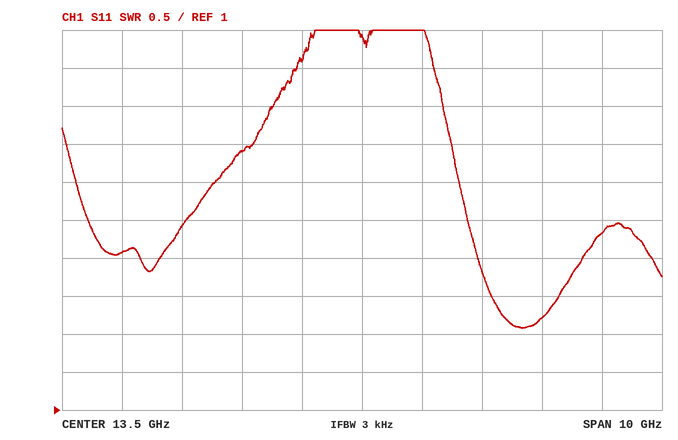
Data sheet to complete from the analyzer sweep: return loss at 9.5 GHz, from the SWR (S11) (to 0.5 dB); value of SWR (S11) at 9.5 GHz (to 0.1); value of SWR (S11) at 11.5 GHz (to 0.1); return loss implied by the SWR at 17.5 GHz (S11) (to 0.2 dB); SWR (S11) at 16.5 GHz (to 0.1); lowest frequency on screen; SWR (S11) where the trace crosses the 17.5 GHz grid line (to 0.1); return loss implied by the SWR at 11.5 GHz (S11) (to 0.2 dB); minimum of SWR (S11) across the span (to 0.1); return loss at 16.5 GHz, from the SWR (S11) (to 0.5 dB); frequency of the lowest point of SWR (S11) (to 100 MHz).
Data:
6.0 dB
3.1
4.4
5.4 dB
2.2
8.5 GHz
3.3
4.0 dB
2.1
8.5 dB
16.2 GHz
